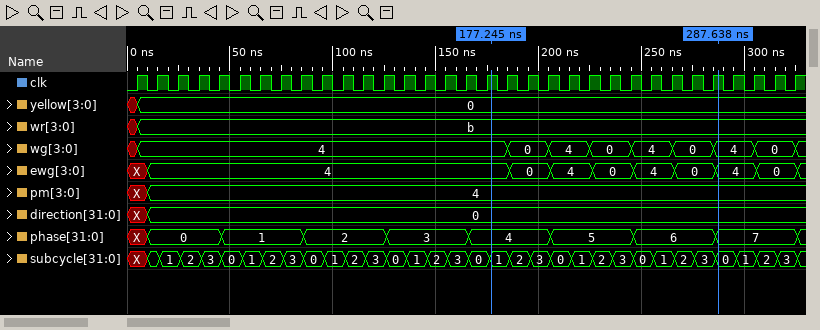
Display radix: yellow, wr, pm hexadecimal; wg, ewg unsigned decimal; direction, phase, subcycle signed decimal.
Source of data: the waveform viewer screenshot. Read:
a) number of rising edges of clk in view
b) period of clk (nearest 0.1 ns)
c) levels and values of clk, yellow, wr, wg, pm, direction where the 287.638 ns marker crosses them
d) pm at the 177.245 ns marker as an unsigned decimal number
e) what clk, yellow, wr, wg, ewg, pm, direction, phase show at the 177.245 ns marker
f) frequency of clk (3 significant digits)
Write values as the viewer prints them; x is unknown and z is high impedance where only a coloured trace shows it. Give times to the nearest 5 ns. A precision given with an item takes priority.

33
10 ns
clk=1, yellow=0, wr=b, wg=4, pm=4, direction=0
4
clk=1, yellow=0, wr=b, wg=4, ewg=4, pm=4, direction=0, phase=4
100 MHz
